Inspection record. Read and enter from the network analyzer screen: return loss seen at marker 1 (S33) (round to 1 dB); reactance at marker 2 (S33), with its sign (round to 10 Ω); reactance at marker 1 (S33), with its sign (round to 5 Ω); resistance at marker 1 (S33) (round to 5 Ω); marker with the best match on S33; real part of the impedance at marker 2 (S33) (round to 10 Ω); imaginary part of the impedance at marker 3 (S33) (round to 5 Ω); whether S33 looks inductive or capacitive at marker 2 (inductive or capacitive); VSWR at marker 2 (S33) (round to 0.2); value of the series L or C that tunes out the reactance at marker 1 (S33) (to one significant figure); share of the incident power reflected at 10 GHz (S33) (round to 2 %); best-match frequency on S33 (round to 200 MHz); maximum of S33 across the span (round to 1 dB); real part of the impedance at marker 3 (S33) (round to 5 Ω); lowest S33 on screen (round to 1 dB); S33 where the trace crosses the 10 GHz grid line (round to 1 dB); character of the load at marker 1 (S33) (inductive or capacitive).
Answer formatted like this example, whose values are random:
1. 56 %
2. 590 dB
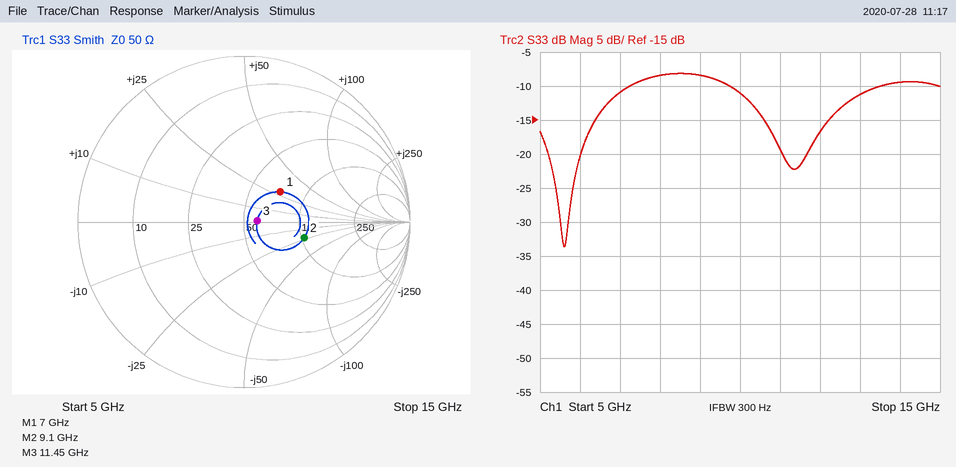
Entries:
1. 11 dB
2. -20 Ω
3. +30 Ω
4. 70 Ω
5. marker 3
6. 100 Ω
7. 0 Ω
8. capacitive
9. 2.2
10. 800 fF
11. 8 %
12. 5.6 GHz
13. -8 dB
14. 60 Ω
15. -34 dB
16. -11 dB
17. inductive
